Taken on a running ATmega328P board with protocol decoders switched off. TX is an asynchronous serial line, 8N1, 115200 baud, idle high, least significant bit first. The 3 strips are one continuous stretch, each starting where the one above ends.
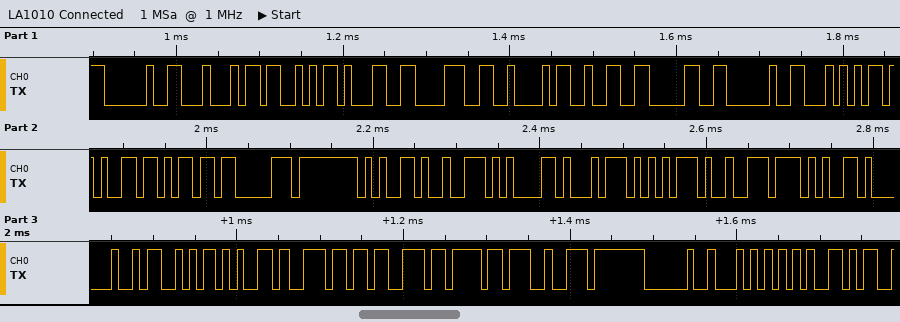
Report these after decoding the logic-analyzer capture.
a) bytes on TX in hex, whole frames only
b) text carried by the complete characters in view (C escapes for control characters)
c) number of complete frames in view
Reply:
0x20 0x44 0x53 0x31 0x38 0x42 0x32 0x30 0x20 0x54 0x65 0x6D 0x70 0x65 0x72 0x61 0x74 0x75 0x72 0x65 0x20 0x53 0x65 0x6E 0x73 0x6F 0x72 0x20 0x54 0x65
" DS18B20 Temperature Sensor Te"
30
